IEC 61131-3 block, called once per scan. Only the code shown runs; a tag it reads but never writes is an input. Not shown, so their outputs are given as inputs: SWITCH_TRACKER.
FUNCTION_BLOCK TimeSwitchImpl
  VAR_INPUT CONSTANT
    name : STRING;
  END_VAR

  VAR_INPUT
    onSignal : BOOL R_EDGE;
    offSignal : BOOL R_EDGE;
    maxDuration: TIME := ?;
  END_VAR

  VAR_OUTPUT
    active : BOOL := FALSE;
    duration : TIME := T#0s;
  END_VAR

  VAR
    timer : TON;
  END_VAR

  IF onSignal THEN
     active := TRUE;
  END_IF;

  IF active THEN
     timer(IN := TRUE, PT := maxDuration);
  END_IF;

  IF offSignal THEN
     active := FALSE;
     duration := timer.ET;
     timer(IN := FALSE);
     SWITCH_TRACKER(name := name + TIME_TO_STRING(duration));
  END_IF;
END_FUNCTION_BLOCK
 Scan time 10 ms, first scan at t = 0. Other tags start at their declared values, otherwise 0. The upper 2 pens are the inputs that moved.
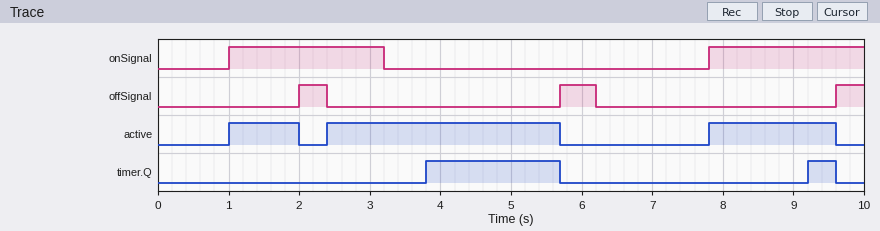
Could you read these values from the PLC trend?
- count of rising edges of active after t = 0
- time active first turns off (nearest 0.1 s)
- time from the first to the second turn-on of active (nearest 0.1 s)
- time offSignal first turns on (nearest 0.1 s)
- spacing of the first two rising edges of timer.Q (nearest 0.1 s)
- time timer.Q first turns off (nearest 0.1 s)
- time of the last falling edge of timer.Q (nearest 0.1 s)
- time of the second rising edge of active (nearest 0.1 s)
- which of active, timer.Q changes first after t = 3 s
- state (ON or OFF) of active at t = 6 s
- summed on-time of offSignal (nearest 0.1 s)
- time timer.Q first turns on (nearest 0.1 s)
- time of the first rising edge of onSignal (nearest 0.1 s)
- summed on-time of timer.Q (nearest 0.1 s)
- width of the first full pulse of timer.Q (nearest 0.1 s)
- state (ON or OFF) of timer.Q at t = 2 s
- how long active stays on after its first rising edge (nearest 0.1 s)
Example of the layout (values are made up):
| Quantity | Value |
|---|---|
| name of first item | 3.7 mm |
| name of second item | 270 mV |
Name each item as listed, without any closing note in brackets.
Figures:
| Quantity | Value |
|---|---|
| count of rising edges of active after t = 0 | 3 |
| time active first turns off | 2.0 s |
| time from the first to the second turn-on of active | 1.4 s |
| time offSignal first turns on | 2.0 s |
| spacing of the first two rising edges of timer.Q | 5.4 s |
| time timer.Q first turns off | 5.7 s |
| time of the last falling edge of timer.Q | 9.6 s |
| time of the second rising edge of active | 2.4 s |
| which of active, timer.Q changes first after t = 3 s | timer.Q |
| state (ON or OFF) of active at t = 6 s | OFF |
| summed on-time of offSignal | 1.3 s |
| time timer.Q first turns on | 3.8 s |
| time of the first rising edge of onSignal | 1.0 s |
| summed on-time of timer.Q | 2.3 s |
| width of the first full pulse of timer.Q | 1.9 s |
| state (ON or OFF) of timer.Q at t = 2 s | OFF |
| how long active stays on after its first rising edge | 1.0 s |
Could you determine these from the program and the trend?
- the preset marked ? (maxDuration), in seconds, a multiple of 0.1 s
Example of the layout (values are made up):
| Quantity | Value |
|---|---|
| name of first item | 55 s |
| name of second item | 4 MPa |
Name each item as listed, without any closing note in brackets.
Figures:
| Quantity | Value |
|---|---|
| the preset marked ? (maxDuration), in seconds, a multiple of 0.1 s | 1.4 s |
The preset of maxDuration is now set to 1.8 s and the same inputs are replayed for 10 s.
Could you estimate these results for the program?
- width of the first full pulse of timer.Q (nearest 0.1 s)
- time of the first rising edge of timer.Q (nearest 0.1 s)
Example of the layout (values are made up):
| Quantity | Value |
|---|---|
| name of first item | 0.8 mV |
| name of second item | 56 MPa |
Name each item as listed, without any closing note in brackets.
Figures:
| Quantity | Value |
|---|---|
| width of the first full pulse of timer.Q | 1.5 s |
| time of the first rising edge of timer.Q | 4.2 s |
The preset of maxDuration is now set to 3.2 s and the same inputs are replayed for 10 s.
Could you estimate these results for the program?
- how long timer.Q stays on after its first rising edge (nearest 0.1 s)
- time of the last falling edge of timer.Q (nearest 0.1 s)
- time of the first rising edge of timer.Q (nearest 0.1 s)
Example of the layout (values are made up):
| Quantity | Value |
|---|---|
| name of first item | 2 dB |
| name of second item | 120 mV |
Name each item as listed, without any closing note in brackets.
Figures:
| Quantity | Value |
|---|---|
| how long timer.Q stays on after its first rising edge | 0.1 s |
| time of the last falling edge of timer.Q | 5.7 s |
| time of the first rising edge of timer.Q | 5.6 s |
